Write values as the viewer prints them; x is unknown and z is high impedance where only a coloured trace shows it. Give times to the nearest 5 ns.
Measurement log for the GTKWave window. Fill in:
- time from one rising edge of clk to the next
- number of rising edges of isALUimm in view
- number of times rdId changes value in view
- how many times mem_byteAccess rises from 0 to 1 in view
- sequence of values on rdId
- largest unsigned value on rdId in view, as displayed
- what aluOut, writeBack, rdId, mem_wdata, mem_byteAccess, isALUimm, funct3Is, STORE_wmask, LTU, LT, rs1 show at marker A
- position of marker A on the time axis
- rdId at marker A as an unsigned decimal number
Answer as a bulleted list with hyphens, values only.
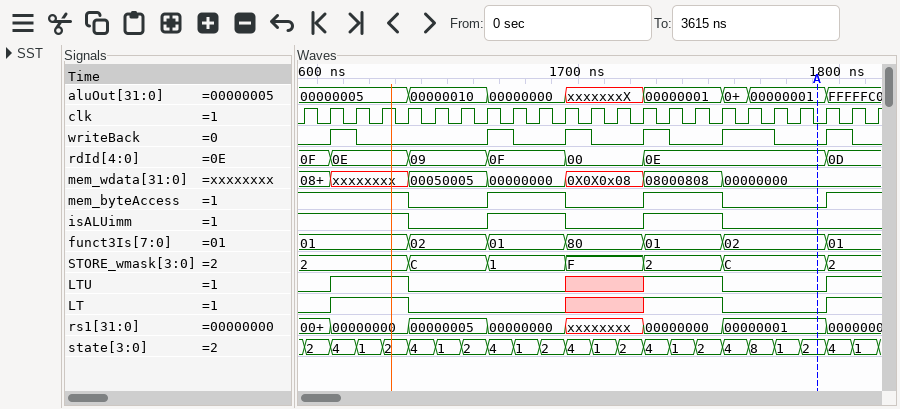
- 10 ns
- 2
- 6
- 3
- 0F, 0E, 09, 0F, 00, 0E, 0D
- 0F
- aluOut=00000001, writeBack=0, rdId=0E, mem_wdata=00000000, mem_byteAccess=0, isALUimm=0, funct3Is=02, STORE_wmask=C, LTU=0, LT=0, rs1=00000001
- 1790 ns
- 14
